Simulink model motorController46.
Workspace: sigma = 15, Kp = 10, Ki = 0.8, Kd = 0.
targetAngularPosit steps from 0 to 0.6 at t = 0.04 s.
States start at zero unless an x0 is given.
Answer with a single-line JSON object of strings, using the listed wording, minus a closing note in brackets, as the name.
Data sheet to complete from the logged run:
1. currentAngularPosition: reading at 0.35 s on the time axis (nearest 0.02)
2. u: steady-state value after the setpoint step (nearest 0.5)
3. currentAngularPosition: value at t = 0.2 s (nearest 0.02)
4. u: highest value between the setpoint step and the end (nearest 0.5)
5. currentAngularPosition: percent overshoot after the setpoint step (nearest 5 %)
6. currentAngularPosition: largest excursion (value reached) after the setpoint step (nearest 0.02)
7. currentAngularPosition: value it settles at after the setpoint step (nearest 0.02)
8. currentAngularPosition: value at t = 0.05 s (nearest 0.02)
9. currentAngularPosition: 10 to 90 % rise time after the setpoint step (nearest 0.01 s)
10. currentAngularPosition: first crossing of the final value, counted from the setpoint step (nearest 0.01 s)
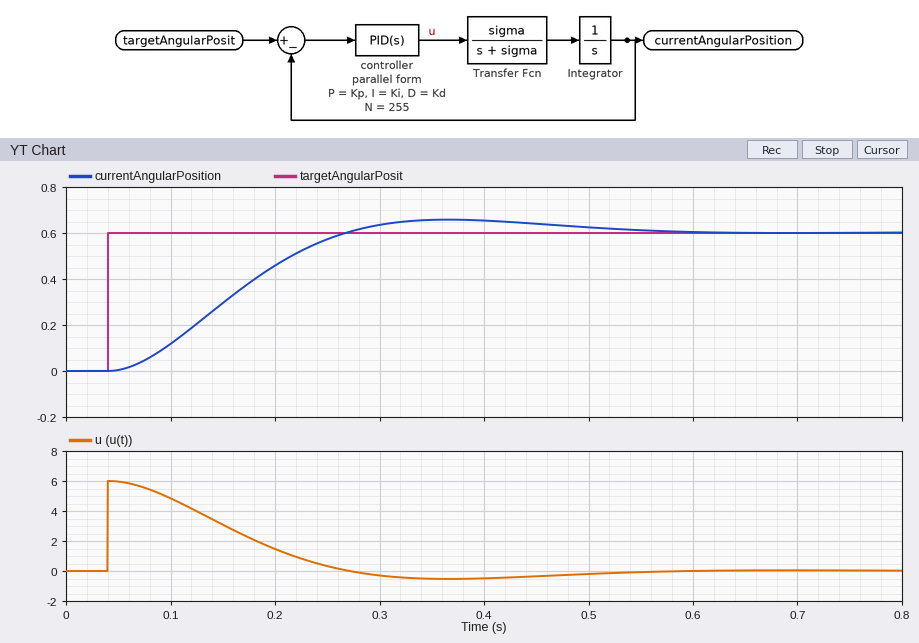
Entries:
{"currentAngularPosition: reading at 0.35 s on the time axis": "0.66", "u: steady-state value after the setpoint step": "0.0", "currentAngularPosition: value at t = 0.2 s": "0.46", "u: highest value between the setpoint step and the end": "6.0", "currentAngularPosition: percent overshoot after the setpoint step": "10 %", "currentAngularPosition: largest excursion (value reached) after the setpoint step": "0.66", "currentAngularPosition: value it settles at after the setpoint step": "0.60", "currentAngularPosition: value at t = 0.05 s": "0.00", "currentAngularPosition: 10 to 90 % rise time after the setpoint step": "0.15 s", "currentAngularPosition: first crossing of the final value, counted from the setpoint step": "0.23 s"}
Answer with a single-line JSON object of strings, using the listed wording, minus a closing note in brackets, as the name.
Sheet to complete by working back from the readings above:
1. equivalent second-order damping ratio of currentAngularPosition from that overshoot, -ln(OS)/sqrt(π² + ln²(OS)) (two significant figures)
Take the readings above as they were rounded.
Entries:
{"equivalent second-order damping ratio of currentAngularPosition from that overshoot, -ln(OS)/sqrt(π² + ln²(OS))": "0.59"}
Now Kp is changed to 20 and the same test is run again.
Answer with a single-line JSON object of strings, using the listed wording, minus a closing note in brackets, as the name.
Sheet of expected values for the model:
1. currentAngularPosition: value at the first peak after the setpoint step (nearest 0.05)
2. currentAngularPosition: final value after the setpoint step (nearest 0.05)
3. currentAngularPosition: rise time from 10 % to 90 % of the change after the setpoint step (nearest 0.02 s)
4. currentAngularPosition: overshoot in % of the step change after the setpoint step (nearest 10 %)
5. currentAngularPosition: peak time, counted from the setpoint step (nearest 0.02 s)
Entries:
{"currentAngularPosition: value at the first peak after the setpoint step": "0.75", "currentAngularPosition: final value after the setpoint step": "0.60", "currentAngularPosition: rise time from 10 % to 90 % of the change after the setpoint step": "0.08 s", "currentAngularPosition: overshoot in % of the step change after the setpoint step": "20 %", "currentAngularPosition: peak time, counted from the setpoint step": "0.20 s"}
